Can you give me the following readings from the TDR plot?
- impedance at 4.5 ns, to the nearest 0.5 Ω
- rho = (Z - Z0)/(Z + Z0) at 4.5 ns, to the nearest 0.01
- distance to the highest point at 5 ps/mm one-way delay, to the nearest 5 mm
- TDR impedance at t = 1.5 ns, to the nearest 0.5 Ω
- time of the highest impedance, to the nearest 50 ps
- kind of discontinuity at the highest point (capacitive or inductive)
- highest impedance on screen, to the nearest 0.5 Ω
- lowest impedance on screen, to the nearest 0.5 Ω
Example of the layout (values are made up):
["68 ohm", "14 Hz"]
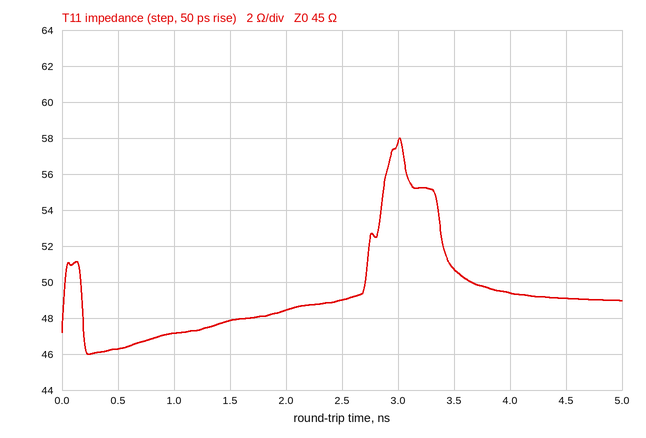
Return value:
["49.0 Ω", "+0.04", "300 mm", "48.0 Ω", "3.00 ns", "inductive", "58.0 Ω", "46.0 Ω"]
